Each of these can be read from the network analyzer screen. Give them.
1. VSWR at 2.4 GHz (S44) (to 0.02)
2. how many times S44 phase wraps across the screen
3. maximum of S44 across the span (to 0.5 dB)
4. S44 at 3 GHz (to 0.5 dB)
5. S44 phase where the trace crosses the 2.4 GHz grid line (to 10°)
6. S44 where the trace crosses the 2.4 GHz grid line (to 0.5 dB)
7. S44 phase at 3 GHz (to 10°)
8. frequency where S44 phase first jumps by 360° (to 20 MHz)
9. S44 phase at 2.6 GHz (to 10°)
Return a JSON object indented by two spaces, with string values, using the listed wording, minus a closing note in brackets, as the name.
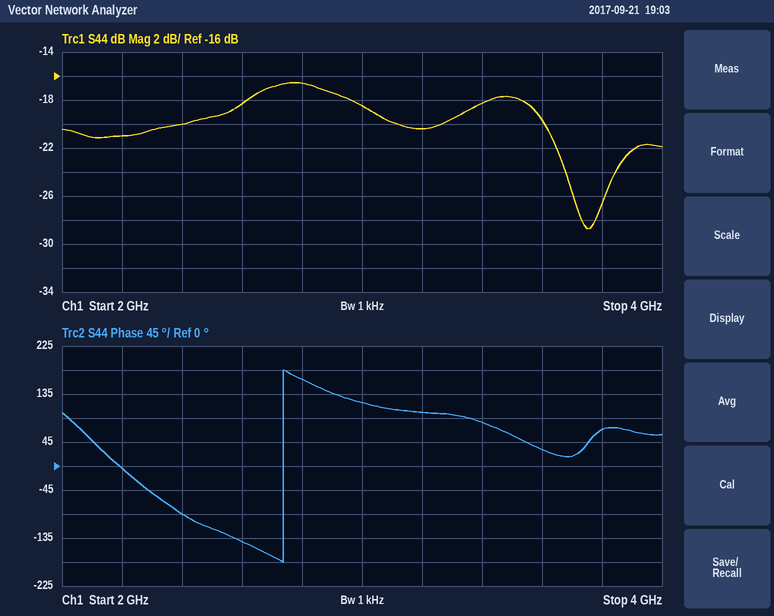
{
  "VSWR at 2.4 GHz (S44)": "1.22",
  "how many times S44 phase wraps across the screen": "1",
  "maximum of S44 across the span": "-16.5 dB",
  "S44 at 3 GHz": "-18.5 dB",
  "S44 phase where the trace crosses the 2.4 GHz grid line": "-90°",
  "S44 where the trace crosses the 2.4 GHz grid line": "-20.0 dB",
  "S44 phase at 3 GHz": "120°",
  "frequency where S44 phase first jumps by 360°": "2.74 GHz",
  "S44 phase at 2.6 GHz": "-140°"
}
